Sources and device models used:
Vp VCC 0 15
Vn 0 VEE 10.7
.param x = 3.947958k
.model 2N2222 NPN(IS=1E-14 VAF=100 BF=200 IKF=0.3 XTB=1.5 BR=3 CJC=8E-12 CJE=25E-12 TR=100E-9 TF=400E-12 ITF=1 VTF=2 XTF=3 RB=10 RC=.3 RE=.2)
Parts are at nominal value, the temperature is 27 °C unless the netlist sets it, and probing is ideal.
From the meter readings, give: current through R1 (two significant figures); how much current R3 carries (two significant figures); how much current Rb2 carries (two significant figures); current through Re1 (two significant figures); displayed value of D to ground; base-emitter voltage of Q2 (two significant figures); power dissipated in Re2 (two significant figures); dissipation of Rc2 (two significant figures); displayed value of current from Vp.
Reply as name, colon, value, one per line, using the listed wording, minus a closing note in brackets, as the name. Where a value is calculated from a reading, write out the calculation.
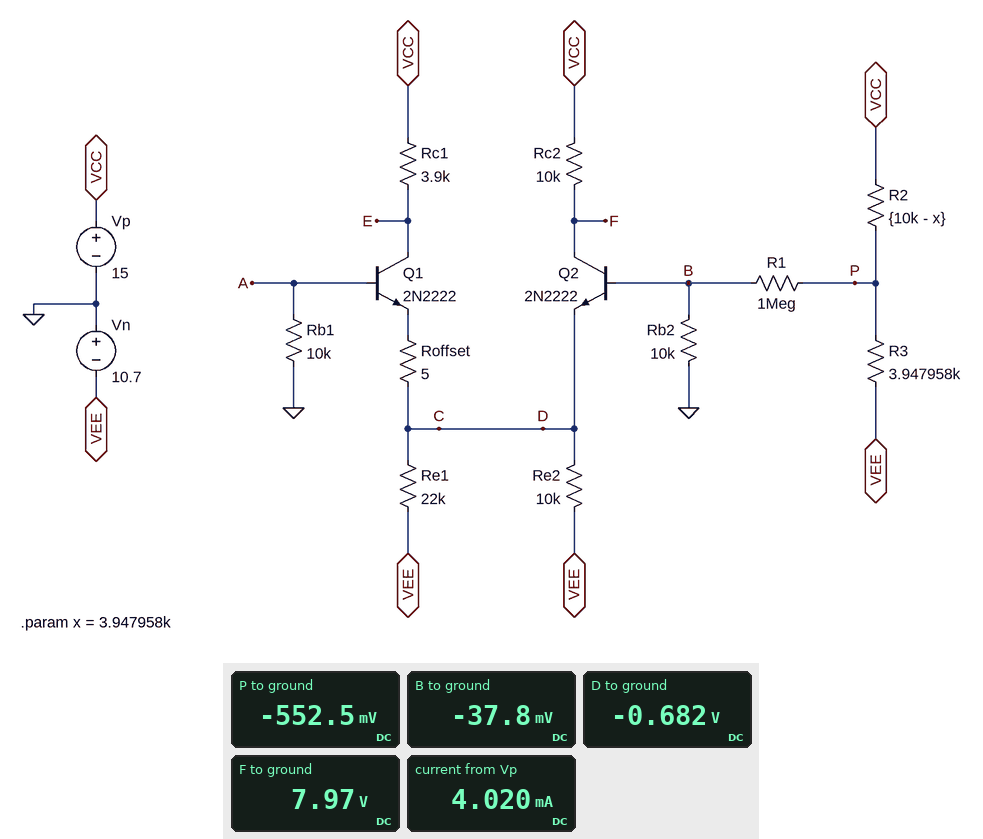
current through R1: (-37.8 mV - (-552.5 mV)) / 1 MΩ = 510 nA
how much current R3 carries: (-552.5 mV - (-10.7 V)) / 3.948 kΩ = 2.6 mA
how much current Rb2 carries: (0 V - (-37.8 mV)) / 10 kΩ = 3.8 µA
current through Re1: (-682 mV - (-10.7 V)) / 22 kΩ = 460 µA
displayed value of D to ground: -0.682 V
base-emitter voltage of Q2: -37.8 mV - (-682 mV) = 640 mV
power dissipated in Re2: (-682 mV - (-10.7 V))^2 / 10 kΩ = 10 mW
dissipation of Rc2: (15 V - 7.97 V)^2 / 10 kΩ = 4.9 mW
displayed value of current from Vp: 4.020 mA
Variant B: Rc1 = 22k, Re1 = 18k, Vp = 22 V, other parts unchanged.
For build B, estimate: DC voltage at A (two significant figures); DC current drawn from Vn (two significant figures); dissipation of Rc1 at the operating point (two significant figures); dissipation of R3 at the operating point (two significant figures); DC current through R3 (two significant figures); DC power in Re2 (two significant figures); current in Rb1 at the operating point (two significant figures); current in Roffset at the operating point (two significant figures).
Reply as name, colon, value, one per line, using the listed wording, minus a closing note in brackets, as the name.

DC voltage at A: -28 mV
DC current drawn from Vn: 4.8 mA
dissipation of Rc1 at the operating point: 8.0 mW
dissipation of R3 at the operating point: 42 mW
DC current through R3: 3.3 mA
DC power in Re2: 10 mW
current in Rb1 at the operating point: 2.8 µA
current in Roffset at the operating point: 610 µA
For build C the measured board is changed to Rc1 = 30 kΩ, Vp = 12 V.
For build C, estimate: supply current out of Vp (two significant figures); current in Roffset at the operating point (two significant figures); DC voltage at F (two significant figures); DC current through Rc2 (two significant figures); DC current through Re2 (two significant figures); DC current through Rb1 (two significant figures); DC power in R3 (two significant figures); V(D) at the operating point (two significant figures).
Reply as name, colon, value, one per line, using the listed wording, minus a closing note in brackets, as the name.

supply current out of Vp: 3.7 mA
current in Roffset at the operating point: 430 µA
DC voltage at F: 1.8 V
DC current through Rc2: 1.0 mA
DC current through Re2: 1.0 mA
DC current through Rb1: 8.5 µA
DC power in R3: 20 mW
V(D) at the operating point: -720 mV
